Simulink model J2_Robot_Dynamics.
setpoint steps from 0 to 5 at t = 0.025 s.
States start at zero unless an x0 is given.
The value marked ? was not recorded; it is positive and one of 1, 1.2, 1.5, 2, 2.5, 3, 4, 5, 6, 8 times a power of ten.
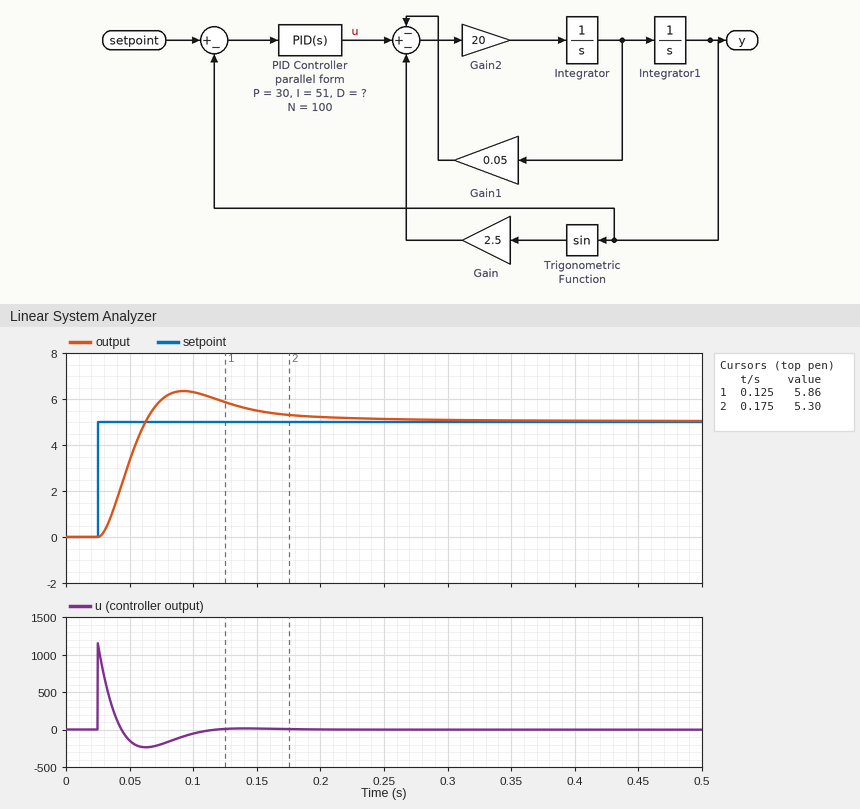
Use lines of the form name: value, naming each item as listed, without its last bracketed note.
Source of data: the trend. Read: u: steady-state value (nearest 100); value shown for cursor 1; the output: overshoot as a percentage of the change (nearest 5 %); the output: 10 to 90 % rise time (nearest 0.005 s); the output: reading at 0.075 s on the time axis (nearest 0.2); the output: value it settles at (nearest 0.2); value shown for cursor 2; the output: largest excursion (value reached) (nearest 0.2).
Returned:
u: steady-state value: 0
value shown for cursor 1: 5.86
the output: overshoot as a percentage of the change: 25 %
the output: 10 to 90 % rise time: 0.025 s
the output: reading at 0.075 s on the time axis: 6.0
the output: value it settles at: 5.0
value shown for cursor 2: 5.30
the output: largest excursion (value reached): 6.4
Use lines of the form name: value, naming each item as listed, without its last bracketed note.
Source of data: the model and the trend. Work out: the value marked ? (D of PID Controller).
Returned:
the value marked ?: 2
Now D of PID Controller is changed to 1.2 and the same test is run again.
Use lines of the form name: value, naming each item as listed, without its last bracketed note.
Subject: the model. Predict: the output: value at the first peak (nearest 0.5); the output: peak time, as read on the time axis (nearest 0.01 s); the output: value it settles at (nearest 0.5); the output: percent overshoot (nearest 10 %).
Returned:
the output: value at the first peak: 7.0
the output: peak time, as read on the time axis: 0.11 s
the output: value it settles at: 5.0
the output: percent overshoot: 40 %
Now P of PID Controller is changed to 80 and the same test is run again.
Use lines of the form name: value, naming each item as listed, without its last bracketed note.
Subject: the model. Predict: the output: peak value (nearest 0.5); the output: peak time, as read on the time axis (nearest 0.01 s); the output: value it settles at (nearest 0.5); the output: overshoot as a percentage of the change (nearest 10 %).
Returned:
the output: peak value: 7.5
the output: peak time, as read on the time axis: 0.08 s
the output: value it settles at: 5.0
the output: overshoot as a percentage of the change: 50 %
